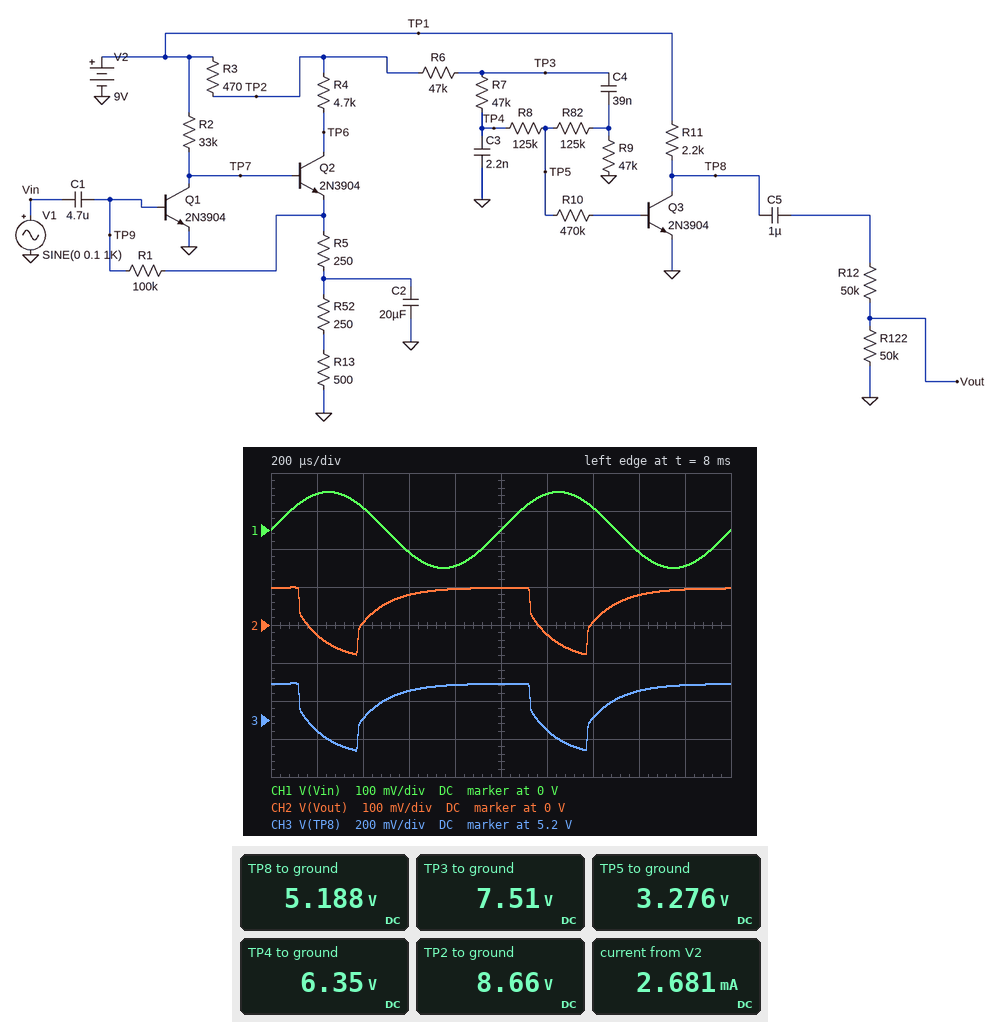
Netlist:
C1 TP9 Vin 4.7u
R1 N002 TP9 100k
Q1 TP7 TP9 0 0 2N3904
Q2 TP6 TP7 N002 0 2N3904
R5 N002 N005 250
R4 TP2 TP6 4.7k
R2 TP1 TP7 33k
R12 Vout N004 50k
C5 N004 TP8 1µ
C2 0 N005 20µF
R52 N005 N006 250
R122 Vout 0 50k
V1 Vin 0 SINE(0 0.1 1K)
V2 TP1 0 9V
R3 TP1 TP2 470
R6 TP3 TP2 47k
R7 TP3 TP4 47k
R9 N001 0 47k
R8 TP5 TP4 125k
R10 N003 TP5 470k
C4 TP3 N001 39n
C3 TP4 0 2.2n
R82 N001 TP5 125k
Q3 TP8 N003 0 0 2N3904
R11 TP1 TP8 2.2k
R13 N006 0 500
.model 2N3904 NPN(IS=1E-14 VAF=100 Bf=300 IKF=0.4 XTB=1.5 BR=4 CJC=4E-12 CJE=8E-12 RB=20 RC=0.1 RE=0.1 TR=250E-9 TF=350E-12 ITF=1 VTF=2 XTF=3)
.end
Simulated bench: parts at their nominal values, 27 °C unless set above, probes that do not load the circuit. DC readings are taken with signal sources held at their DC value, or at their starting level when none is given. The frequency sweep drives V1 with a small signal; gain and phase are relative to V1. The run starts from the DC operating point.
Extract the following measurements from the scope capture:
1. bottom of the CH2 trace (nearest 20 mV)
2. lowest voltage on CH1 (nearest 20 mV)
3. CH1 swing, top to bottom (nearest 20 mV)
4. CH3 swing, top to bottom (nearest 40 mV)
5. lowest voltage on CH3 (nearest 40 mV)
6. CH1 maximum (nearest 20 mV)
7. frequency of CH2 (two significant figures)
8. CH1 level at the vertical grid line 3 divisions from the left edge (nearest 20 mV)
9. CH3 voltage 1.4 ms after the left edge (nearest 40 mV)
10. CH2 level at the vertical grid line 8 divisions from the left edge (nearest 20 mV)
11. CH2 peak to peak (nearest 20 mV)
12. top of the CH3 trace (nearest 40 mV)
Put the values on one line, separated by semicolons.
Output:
-80 mV; -100 mV; 200 mV; 360 mV; 5.04 V; 100 mV; 1.0 kHz; -60 mV; 5.20 V; 80 mV; 180 mV; 5.40 V
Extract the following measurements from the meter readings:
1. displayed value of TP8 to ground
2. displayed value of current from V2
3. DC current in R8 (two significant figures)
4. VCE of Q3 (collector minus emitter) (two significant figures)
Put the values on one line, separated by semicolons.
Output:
5.188 V; 2.681 mA; 25 µA; 5.2 V
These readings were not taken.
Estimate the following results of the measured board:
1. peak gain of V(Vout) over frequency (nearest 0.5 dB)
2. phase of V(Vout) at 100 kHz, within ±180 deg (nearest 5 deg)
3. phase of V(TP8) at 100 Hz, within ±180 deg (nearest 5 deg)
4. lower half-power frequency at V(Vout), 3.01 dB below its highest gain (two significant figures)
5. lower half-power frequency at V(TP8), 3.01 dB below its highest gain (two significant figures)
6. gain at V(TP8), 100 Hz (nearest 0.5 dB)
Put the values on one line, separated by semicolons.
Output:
38.5 dB; 100 deg; -135 deg; 66 Hz; 66 Hz; 43.5 dB
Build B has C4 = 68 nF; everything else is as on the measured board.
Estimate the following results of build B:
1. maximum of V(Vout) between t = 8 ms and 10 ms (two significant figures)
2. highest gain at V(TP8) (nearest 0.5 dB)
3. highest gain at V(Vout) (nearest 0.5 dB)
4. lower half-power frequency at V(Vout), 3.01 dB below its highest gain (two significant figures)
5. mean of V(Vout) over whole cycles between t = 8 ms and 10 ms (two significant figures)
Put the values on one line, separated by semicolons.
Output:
100 mV; 45.0 dB; 39.0 dB; 65 Hz; 50 mV
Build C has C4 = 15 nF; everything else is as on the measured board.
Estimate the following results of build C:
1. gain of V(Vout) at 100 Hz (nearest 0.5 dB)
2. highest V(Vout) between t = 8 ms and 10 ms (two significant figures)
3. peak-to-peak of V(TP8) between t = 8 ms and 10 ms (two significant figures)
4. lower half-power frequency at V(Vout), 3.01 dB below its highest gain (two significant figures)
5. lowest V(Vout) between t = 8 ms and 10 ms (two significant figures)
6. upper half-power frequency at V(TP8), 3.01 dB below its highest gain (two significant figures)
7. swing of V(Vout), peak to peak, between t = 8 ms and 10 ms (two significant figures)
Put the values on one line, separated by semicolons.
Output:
37.0 dB; 96 mV; 340 mV; 67 Hz; -74 mV; 1.6 kHz; 170 mV
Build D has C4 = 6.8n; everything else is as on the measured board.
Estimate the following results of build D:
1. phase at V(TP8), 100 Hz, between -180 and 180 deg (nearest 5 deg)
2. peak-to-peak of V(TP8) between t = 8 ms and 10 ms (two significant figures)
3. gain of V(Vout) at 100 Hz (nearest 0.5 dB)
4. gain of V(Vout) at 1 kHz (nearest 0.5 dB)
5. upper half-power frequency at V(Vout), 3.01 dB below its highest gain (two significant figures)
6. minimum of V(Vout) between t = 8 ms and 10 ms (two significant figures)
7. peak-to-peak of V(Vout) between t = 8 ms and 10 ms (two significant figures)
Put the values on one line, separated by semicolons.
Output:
-140 deg; 320 mV; 37.0 dB; 36.5 dB; 1.6 kHz; -67 mV; 160 mV
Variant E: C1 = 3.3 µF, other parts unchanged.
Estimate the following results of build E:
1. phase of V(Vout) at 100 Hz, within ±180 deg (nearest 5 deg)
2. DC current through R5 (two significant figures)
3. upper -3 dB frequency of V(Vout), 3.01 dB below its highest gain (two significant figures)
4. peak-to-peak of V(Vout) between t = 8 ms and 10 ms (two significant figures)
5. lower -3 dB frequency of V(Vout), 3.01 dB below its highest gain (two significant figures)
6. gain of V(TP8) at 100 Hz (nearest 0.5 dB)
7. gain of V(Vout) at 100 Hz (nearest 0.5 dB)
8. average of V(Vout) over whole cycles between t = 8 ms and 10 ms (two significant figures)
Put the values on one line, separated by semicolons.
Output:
-125 deg; 690 µA; 1.6 kHz; 170 mV; 84 Hz; 42.5 dB; 36.5 dB; 52 mV
